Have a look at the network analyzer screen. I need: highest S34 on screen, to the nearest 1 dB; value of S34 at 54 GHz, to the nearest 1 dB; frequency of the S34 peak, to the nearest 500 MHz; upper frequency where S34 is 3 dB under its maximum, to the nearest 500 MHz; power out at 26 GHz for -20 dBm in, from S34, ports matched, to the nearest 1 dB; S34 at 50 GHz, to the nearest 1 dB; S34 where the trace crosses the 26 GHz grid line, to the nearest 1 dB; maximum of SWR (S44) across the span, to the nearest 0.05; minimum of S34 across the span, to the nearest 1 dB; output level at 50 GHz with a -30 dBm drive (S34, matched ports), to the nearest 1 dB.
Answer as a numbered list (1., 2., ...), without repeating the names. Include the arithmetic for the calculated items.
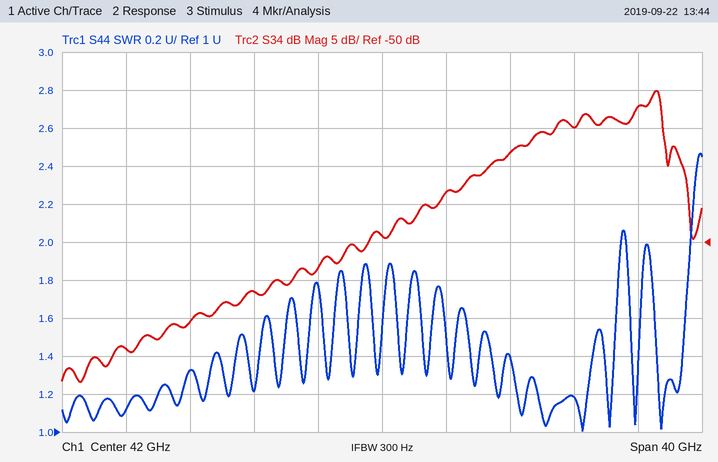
1. -30 dB
2. -35 dB
3. 59.0 GHz
4. 59.5 GHz
5. -20 dBm + (-64 dB) = -84 dBm
6. -38 dB
7. -64 dB
8. 2.45
9. -68 dB
10. -30 dBm + (-38 dB) = -68 dBm
